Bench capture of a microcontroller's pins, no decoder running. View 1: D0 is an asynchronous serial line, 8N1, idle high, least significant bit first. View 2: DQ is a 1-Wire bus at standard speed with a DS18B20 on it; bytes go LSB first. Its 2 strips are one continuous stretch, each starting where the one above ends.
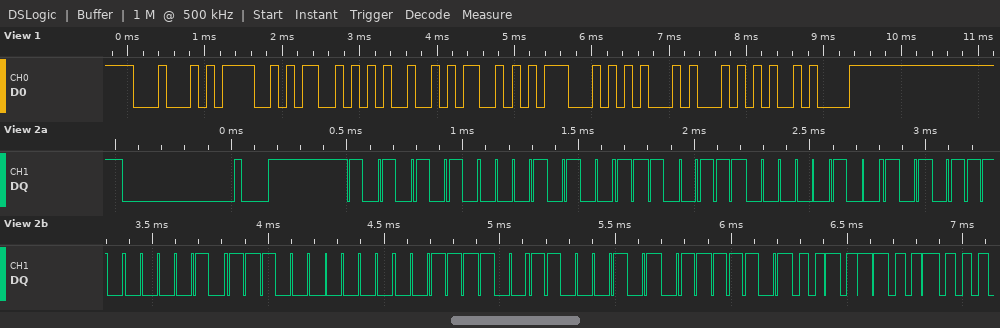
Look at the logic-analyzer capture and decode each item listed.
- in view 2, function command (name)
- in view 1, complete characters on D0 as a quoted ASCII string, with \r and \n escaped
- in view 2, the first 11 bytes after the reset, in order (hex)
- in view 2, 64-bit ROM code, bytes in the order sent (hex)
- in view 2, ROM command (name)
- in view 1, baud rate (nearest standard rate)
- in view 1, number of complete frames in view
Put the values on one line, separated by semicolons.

Read Scratchpad; "DOSISGET\n"; 55 28 E7 20 75 D0 01 3C A3 BE 34; 28 E7 20 75 D0 01 3C A3; Match ROM; 9600 baud; 9
